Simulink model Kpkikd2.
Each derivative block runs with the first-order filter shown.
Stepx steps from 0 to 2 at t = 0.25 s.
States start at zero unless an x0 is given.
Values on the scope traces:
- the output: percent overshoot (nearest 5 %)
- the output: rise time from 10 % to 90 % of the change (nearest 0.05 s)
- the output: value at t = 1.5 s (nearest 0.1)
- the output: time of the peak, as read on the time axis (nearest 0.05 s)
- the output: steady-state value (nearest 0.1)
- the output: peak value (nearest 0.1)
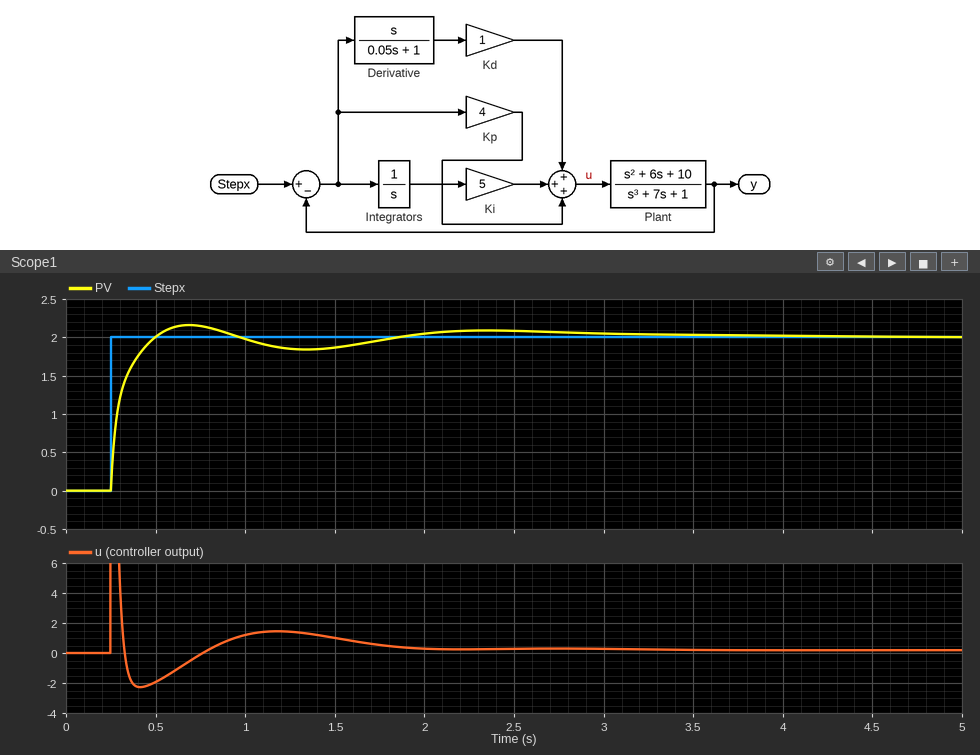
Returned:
10 %
0.15 s
1.9
0.70 s
2.0
2.2
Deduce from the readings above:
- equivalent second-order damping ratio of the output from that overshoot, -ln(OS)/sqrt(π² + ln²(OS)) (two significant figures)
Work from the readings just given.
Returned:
0.59
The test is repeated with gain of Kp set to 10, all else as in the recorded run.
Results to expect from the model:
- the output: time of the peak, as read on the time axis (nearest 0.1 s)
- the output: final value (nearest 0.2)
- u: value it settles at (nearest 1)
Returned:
0.6 s
2.0
0
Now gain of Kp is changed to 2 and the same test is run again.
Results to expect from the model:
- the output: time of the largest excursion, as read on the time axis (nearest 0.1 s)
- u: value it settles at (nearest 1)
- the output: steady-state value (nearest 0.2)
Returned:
2.5 s
0
2.0
